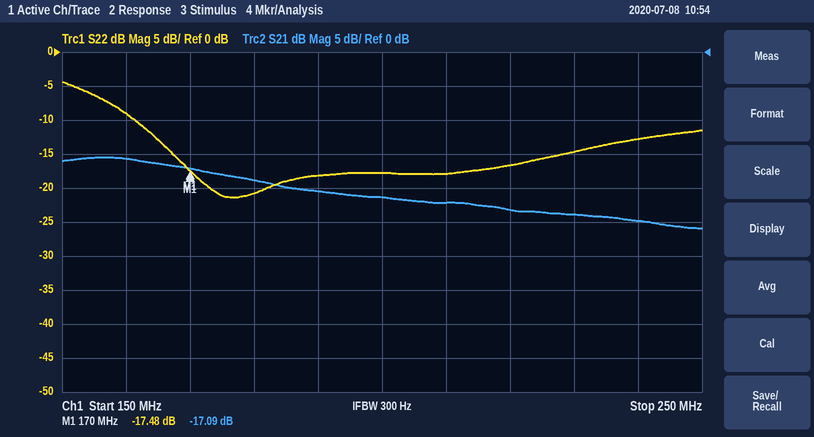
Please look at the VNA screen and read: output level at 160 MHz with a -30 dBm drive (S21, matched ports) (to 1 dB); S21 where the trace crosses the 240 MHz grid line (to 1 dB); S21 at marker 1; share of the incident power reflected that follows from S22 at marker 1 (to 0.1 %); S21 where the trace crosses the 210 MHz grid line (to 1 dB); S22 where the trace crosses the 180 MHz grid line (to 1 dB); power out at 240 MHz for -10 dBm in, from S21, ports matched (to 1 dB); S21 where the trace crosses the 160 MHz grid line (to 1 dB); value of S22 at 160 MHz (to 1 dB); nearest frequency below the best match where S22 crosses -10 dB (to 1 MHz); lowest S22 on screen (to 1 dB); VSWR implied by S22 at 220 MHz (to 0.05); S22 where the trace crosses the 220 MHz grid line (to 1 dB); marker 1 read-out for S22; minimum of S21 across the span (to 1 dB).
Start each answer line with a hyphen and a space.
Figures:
- -46 dBm
- -25 dB
- -17.09 dB
- 1.8 %
- -22 dB
- -21 dB
- -35 dBm
- -16 dB
- -9 dB
- 161 MHz
- -21 dB
- 1.35
- -17 dB
- -17.48 dB
- -26 dB
